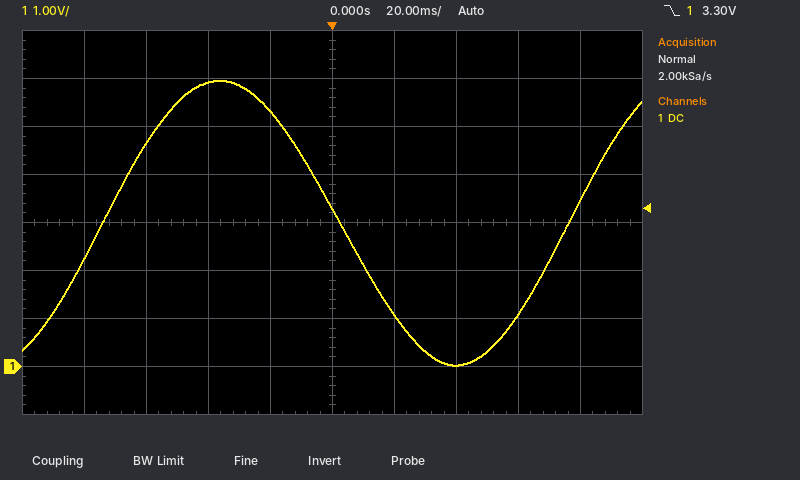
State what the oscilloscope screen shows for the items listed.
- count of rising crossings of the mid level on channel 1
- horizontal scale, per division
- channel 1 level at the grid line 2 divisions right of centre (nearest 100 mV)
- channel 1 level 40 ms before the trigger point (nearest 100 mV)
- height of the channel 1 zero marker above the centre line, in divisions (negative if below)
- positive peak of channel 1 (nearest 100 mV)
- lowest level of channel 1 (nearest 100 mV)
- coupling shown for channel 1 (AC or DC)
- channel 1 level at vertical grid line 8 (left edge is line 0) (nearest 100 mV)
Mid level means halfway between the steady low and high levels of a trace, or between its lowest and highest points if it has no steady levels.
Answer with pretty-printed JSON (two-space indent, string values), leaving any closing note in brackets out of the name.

{
  "count of rising crossings of the mid level on channel 1": "2",
  "horizontal scale, per division": "20 ms",
  "channel 1 level at the grid line 2 divisions right of centre": "0.0 V",
  "channel 1 level 40 ms before the trigger point": "5.9 V",
  "height of the channel 1 zero marker above the centre line, in divisions": "-3.0 div",
  "positive peak of channel 1": "6.0 V",
  "lowest level of channel 1": "0.0 V",
  "coupling shown for channel 1": "DC",
  "channel 1 level at vertical grid line 8 (left edge is line 0)": "1.1 V"
}
